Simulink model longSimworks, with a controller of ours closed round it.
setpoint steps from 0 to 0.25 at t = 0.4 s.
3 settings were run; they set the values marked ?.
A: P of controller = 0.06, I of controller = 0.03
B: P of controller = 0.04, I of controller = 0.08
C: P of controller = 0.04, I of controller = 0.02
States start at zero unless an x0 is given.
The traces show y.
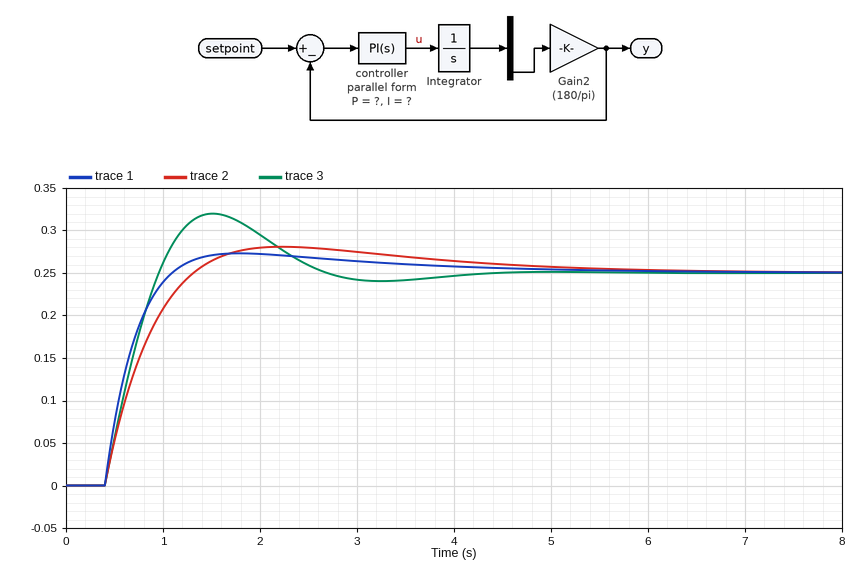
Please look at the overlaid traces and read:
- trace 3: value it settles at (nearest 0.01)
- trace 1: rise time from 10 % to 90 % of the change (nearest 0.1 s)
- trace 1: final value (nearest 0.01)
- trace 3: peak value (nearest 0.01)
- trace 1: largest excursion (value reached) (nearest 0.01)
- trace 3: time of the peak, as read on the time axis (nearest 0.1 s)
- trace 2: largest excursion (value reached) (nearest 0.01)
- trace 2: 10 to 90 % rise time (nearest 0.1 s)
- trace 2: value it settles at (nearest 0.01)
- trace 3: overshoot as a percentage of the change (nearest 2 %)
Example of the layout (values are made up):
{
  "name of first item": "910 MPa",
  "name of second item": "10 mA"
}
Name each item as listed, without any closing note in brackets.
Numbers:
{
  "trace 3: value it settles at": "0.25",
  "trace 1: rise time from 10 % to 90 % of the change": "0.5 s",
  "trace 1: final value": "0.25",
  "trace 3: peak value": "0.32",
  "trace 1: largest excursion (value reached)": "0.27",
  "trace 3: time of the peak, as read on the time axis": "1.5 s",
  "trace 2: largest excursion (value reached)": "0.28",
  "trace 2: 10 to 90 % rise time": "0.7 s",
  "trace 2: value it settles at": "0.25",
  "trace 3: overshoot as a percentage of the change": "28 %"
}
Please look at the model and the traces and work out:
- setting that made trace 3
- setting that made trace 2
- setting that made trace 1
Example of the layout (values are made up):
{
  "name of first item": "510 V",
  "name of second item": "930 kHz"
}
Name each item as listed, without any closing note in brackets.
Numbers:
{
  "setting that made trace 3": "B",
  "setting that made trace 2": "C",
  "setting that made trace 1": "A"
}
